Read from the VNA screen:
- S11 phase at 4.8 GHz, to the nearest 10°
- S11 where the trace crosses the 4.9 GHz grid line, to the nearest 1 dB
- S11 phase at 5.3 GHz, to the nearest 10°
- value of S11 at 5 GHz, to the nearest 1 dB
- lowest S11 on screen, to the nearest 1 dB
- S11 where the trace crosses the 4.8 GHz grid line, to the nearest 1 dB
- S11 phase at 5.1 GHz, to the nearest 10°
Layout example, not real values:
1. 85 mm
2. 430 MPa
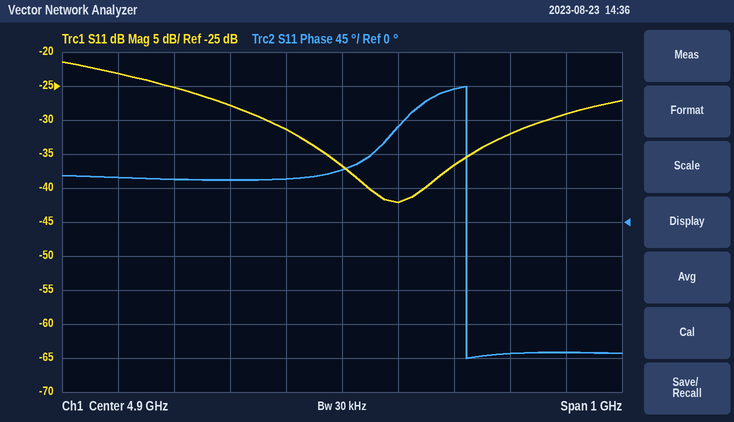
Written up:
1. 60°
2. -37 dB
3. -170°
4. -42 dB
5. -42 dB
6. -31 dB
7. 180°
